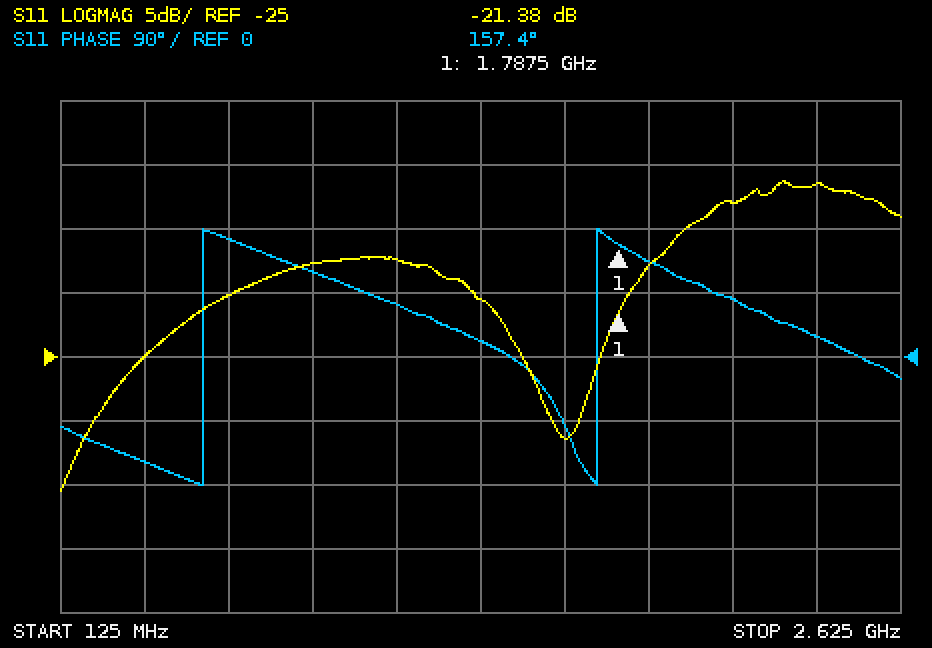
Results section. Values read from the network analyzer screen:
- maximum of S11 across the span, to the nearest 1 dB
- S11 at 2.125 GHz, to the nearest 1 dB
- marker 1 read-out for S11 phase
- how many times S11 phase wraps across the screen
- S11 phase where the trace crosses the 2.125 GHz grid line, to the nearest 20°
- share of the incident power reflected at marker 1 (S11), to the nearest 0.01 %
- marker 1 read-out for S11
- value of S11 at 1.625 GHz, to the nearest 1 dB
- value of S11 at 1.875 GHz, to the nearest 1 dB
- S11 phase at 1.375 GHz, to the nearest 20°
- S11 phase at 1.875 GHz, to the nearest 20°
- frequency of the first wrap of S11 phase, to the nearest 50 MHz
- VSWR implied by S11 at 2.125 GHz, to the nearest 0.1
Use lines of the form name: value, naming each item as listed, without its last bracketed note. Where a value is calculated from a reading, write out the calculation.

maximum of S11 across the span, to the nearest 1 dB: -11 dB
S11 at 2.125 GHz, to the nearest 1 dB: -13 dB
marker 1 read-out for S11 phase: 157.4°
how many times S11 phase wraps across the screen: 2
S11 phase where the trace crosses the 2.125 GHz grid line, to the nearest 20°: 80°
share of the incident power reflected at marker 1 (S11), to the nearest 0.01 %: 10^(-21.38/10) ≈ 0.73 %
marker 1 read-out for S11: -21.38 dB
value of S11 at 1.625 GHz, to the nearest 1 dB: -31 dB
value of S11 at 1.875 GHz, to the nearest 1 dB: -18 dB
S11 phase at 1.375 GHz, to the nearest 20°: 20°
S11 phase at 1.875 GHz, to the nearest 20°: 140°
frequency of the first wrap of S11 phase, to the nearest 50 MHz: 550 MHz
VSWR implied by S11 at 2.125 GHz, to the nearest 0.1: |Γ| = 10^(-13/20) = 0.2239; VSWR = (1 + 0.2239)/(1 − 0.2239) ≈ 1.6
